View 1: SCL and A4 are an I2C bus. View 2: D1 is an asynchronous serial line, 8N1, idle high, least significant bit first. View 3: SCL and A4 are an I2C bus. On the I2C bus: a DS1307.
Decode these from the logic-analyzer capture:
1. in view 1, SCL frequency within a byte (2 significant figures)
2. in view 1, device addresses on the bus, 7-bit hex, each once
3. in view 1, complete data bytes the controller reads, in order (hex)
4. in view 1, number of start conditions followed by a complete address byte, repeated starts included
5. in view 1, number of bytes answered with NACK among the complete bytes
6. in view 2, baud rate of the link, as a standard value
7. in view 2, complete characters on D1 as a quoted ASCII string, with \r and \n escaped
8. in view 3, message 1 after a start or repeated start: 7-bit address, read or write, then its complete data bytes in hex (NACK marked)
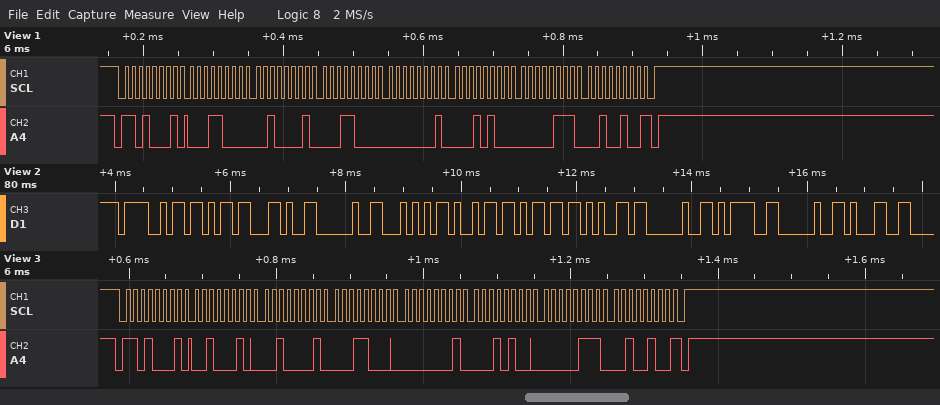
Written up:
100 kHz
0x68
18 21 18 01 14 07 24
1
1
9600 baud
"Ok, Time = 1"
0x68 read: 22 21 18 01 14 07 24 NACK
